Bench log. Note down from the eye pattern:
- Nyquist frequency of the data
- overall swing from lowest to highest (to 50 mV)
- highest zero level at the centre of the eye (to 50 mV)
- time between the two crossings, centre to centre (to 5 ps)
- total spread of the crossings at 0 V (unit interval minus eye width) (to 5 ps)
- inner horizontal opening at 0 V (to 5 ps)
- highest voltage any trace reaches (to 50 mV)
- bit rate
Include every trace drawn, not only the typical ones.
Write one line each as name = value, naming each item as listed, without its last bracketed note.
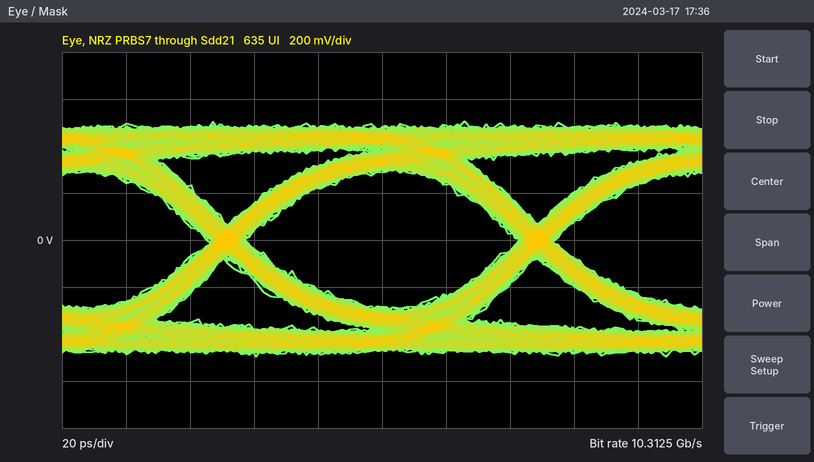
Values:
Nyquist frequency of the data = 5.15625 GHz
overall swing from lowest to highest = 1.00 V
highest zero level at the centre of the eye = -300 mV
time between the two crossings, centre to centre = 95 ps
total spread of the crossings at 0 V (unit interval minus eye width) = 10 ps
inner horizontal opening at 0 V = 85 ps
highest voltage any trace reaches = 500 mV
bit rate = 10.3125 Gb/s
